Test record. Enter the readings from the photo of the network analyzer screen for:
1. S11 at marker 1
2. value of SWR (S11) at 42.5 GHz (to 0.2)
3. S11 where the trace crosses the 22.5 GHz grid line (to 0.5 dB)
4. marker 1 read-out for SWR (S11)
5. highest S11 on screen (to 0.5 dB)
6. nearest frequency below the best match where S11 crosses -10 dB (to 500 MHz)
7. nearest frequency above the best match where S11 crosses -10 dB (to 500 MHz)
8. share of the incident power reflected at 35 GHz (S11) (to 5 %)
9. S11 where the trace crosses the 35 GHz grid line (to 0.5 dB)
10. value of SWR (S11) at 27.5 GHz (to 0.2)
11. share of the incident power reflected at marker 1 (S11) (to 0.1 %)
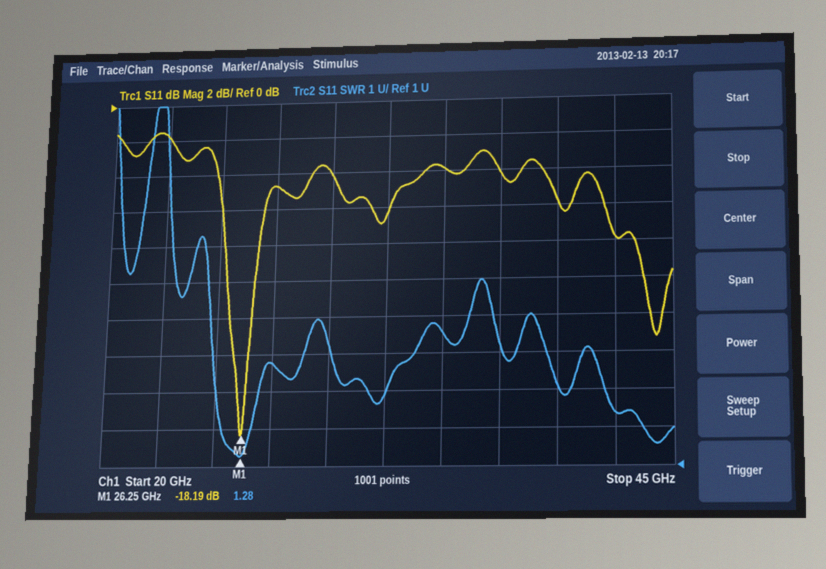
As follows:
-18.19 dB
2.4
-2.0 dB
1.28
-1.5 dB
25.5 GHz
26.5 GHz
40 %
-4.0 dB
3.8
1.5 %
